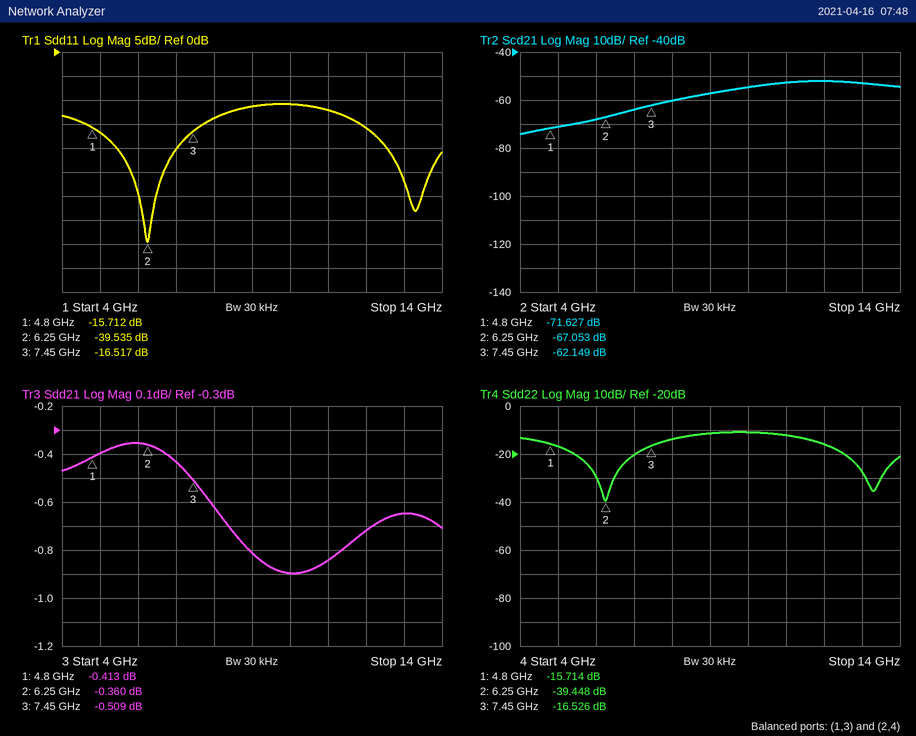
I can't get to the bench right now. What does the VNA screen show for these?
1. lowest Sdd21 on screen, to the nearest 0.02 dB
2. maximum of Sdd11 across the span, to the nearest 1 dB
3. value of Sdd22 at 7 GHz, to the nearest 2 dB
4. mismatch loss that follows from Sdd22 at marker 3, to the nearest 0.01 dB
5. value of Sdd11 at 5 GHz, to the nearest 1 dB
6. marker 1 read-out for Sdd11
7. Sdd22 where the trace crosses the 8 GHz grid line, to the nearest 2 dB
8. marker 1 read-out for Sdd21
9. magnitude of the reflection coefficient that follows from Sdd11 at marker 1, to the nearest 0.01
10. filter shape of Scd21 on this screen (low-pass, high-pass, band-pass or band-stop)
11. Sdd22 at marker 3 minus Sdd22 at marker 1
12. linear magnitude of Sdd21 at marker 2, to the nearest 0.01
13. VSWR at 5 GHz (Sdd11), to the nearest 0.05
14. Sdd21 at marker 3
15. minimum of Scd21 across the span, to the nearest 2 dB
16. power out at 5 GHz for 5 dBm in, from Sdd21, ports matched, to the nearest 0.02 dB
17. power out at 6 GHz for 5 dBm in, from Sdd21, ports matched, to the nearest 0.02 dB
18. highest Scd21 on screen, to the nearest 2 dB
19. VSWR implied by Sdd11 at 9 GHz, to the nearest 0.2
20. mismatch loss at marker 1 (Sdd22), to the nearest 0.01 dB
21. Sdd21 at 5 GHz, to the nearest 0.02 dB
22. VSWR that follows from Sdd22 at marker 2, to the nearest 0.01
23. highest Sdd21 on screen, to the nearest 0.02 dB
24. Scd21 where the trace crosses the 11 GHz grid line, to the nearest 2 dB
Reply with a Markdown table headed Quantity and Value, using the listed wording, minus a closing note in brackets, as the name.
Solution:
| Quantity | Value |
|---|---|
| lowest Sdd21 on screen, to the nearest 0.02 dB | -0.90 dB |
| maximum of Sdd11 across the span, to the nearest 1 dB | -11 dB |
| value of Sdd22 at 7 GHz, to the nearest 2 dB | -20 dB |
| mismatch loss that follows from Sdd22 at marker 3, to the nearest 0.01 dB | 0.10 dB |
| value of Sdd11 at 5 GHz, to the nearest 1 dB | -17 dB |
| marker 1 read-out for Sdd11 | -15.712 dB |
| Sdd22 where the trace crosses the 8 GHz grid line, to the nearest 2 dB | -14 dB |
| marker 1 read-out for Sdd21 | -0.413 dB |
| magnitude of the reflection coefficient that follows from Sdd11 at marker 1, to the nearest 0.01 | 0.16 |
| filter shape of Scd21 on this screen | high-pass |
| Sdd22 at marker 3 minus Sdd22 at marker 1 | -0.812 dB |
| linear magnitude of Sdd21 at marker 2, to the nearest 0.01 | 0.96 |
| VSWR at 5 GHz (Sdd11), to the nearest 0.05 | 1.35 |
| Sdd21 at marker 3 | -0.509 dB |
| minimum of Scd21 across the span, to the nearest 2 dB | -74 dB |
| power out at 5 GHz for 5 dBm in, from Sdd21, ports matched, to the nearest 0.02 dB | 4.60 dBm |
| power out at 6 GHz for 5 dBm in, from Sdd21, ports matched, to the nearest 0.02 dB | 4.64 dBm |
| highest Scd21 on screen, to the nearest 2 dB | -52 dB |
| VSWR implied by Sdd11 at 9 GHz, to the nearest 0.2 | 1.8 |
| mismatch loss at marker 1 (Sdd22), to the nearest 0.01 dB | 0.12 dB |
| Sdd21 at 5 GHz, to the nearest 0.02 dB | -0.40 dB |
| VSWR that follows from Sdd22 at marker 2, to the nearest 0.01 | 1.02 |
| highest Sdd21 on screen, to the nearest 0.02 dB | -0.36 dB |
| Scd21 where the trace crosses the 11 GHz grid line, to the nearest 2 dB | -52 dB |
